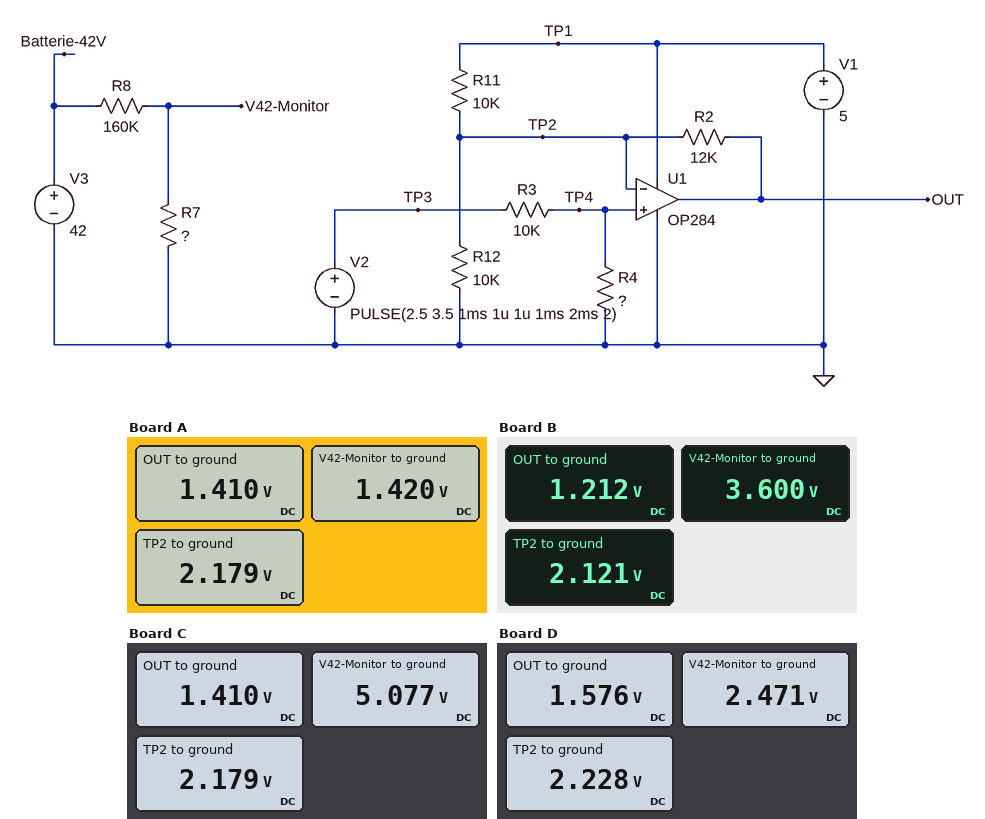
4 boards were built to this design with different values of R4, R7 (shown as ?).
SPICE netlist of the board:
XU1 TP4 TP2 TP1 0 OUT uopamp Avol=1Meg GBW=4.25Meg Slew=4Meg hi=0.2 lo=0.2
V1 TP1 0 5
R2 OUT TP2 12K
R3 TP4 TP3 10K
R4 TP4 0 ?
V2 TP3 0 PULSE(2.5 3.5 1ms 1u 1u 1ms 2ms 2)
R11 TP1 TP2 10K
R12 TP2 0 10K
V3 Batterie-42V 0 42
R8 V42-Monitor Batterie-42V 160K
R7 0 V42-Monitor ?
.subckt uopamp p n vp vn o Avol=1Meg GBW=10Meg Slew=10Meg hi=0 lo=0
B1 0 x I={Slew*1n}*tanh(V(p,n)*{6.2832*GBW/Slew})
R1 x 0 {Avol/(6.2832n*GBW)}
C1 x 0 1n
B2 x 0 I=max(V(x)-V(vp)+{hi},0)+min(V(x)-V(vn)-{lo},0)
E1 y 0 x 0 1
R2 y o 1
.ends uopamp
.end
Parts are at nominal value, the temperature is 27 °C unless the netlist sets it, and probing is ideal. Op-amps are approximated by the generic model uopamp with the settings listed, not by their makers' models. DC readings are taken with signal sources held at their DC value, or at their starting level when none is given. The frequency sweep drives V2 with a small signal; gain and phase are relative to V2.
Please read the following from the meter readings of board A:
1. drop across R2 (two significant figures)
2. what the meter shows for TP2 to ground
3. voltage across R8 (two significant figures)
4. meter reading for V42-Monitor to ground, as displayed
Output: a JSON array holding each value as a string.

["770 mV", "2.179 V", "41 V", "1.420 V"]
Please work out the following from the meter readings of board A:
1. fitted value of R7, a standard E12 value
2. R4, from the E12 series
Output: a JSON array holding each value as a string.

["5.6 kΩ", "68 kΩ"]
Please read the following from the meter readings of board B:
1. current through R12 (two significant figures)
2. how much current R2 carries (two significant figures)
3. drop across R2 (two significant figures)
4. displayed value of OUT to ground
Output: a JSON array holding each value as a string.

["210 µA", "76 µA", "910 mV", "1.212 V"]
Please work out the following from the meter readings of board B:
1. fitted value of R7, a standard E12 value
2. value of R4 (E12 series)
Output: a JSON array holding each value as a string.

["15 kΩ", "56 kΩ"]
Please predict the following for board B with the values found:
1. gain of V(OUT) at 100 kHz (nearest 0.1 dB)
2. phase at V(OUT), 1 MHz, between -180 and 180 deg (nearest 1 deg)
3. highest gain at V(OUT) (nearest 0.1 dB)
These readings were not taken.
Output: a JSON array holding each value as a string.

["9.2 dB", "-39 deg", "9.2 dB"]
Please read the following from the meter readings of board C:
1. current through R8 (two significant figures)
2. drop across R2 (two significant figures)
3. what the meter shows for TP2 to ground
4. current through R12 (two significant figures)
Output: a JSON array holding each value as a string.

["230 µA", "770 mV", "2.179 V", "220 µA"]
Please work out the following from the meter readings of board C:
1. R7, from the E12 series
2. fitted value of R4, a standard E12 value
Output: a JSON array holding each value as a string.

["22 kΩ", "68 kΩ"]
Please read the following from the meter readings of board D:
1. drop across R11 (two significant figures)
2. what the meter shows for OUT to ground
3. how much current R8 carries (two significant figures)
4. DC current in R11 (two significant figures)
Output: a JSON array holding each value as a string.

["2.8 V", "1.576 V", "250 µA", "280 µA"]
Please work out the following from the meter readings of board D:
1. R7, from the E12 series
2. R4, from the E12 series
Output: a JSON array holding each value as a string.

["10 kΩ", "82 kΩ"]
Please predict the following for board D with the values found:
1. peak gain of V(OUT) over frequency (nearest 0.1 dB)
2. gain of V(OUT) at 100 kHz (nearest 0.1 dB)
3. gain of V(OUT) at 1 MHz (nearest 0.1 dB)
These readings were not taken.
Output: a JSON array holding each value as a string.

["9.6 dB", "9.6 dB", "7.5 dB"]
